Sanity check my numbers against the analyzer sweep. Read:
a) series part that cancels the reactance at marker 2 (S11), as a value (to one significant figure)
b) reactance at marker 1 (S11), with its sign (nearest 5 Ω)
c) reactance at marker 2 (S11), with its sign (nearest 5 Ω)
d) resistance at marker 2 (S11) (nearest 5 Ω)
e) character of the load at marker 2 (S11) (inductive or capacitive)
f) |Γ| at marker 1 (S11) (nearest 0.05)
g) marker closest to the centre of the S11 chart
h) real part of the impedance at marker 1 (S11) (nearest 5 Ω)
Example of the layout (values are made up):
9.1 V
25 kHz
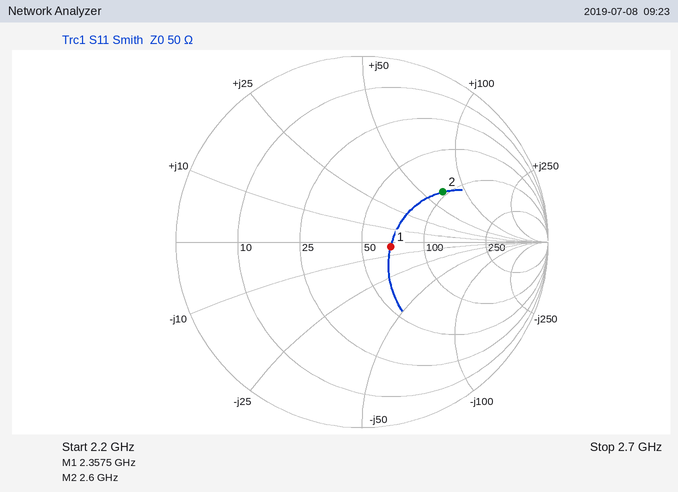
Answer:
900 fF
-5 Ω
+70 Ω
95 Ω
inductive
0.15
marker 1
70 Ω
